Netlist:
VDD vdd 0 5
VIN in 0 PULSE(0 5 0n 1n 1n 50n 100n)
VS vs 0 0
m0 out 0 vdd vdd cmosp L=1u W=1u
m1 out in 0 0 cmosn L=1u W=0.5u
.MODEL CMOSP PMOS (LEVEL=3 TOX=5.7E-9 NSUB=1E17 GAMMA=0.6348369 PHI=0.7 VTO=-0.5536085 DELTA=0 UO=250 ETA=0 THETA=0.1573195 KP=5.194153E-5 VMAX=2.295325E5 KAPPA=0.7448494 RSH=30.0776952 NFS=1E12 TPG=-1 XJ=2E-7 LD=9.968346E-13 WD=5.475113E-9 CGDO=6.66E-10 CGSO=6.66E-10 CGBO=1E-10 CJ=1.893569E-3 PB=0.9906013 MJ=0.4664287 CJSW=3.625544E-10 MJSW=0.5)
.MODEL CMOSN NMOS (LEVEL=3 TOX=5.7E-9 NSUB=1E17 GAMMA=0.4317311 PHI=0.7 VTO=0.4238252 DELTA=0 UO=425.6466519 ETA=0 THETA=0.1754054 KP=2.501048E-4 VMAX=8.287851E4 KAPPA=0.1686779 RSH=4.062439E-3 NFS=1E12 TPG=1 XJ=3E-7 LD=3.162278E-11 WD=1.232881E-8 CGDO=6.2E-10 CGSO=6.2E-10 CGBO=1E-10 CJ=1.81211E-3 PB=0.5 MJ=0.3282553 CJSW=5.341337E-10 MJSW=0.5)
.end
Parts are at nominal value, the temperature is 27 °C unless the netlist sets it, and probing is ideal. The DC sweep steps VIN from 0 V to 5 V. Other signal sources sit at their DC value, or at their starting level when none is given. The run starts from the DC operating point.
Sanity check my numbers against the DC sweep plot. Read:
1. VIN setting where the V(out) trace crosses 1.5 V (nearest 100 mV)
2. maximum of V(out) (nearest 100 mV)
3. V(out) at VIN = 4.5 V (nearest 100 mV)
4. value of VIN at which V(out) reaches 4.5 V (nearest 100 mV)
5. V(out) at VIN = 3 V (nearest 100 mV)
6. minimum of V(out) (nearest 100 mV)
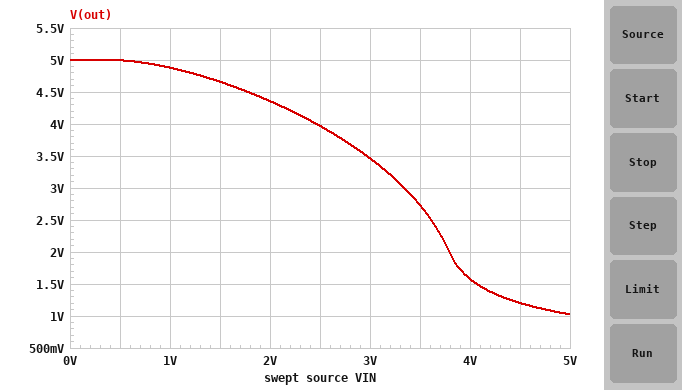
4.1 V
5.0 V
1.2 V
1.8 V
3.5 V
1.0 V
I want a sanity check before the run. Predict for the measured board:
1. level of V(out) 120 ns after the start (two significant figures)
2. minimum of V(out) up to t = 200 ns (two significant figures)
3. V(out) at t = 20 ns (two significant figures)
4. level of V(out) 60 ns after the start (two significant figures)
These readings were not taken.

1.0 V
1.0 V
1.0 V
5.0 V
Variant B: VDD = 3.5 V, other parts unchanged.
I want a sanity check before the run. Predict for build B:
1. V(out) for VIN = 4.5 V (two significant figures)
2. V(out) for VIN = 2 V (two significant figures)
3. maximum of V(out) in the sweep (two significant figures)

490 mV
2.6 V
3.5 V
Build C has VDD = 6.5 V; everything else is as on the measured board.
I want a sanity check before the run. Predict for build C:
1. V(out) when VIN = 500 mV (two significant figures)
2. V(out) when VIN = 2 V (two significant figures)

6.5 V
6.0 V
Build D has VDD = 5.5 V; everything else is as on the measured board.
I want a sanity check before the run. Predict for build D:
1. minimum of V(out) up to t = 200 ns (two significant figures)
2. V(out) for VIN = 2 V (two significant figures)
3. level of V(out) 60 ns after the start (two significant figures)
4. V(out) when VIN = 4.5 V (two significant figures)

1.3 V
4.9 V
5.5 V
1.7 V
